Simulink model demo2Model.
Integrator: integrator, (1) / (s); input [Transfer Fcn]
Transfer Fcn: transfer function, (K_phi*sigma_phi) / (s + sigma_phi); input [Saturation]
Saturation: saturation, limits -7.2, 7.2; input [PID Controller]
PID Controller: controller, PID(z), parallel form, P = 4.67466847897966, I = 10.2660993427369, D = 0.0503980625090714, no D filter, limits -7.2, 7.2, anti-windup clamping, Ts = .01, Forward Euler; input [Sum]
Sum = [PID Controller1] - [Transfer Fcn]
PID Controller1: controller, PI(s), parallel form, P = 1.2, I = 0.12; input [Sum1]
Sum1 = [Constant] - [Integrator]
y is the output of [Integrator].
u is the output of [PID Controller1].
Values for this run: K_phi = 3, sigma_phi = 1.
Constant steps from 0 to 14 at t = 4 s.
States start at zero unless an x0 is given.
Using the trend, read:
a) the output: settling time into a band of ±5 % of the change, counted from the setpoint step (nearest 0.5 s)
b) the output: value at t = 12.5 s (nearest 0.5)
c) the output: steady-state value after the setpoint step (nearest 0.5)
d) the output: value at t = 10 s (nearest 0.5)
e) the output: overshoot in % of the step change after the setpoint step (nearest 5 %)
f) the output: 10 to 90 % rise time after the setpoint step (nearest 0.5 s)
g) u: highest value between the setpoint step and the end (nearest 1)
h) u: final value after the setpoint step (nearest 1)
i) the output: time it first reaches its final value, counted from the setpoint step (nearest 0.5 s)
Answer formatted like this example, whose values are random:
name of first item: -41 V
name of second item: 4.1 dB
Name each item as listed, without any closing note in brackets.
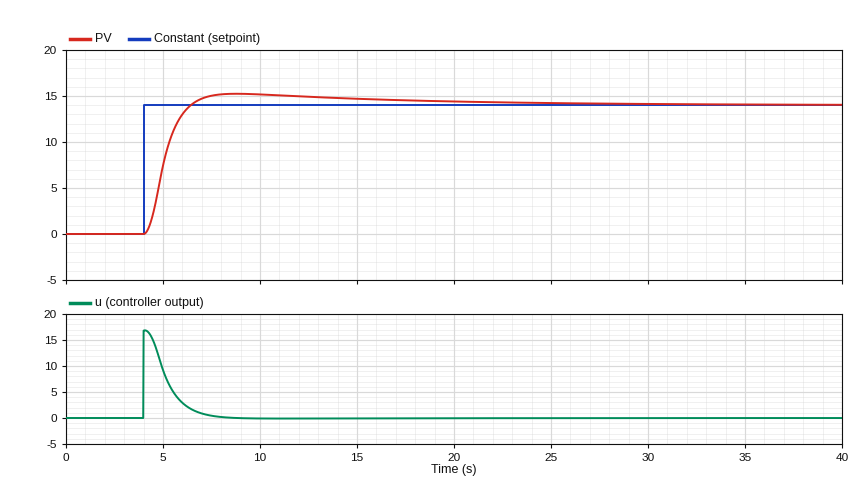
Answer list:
the output: settling time into a band of ±5 % of the change, counted from the setpoint step: 11.0 s
the output: value at t = 12.5 s: 15.0
the output: steady-state value after the setpoint step: 14.0
the output: value at t = 10 s: 15.0
the output: overshoot in % of the step change after the setpoint step: 10 %
the output: 10 to 90 % rise time after the setpoint step: 1.5 s
u: highest value between the setpoint step and the end: 17
u: final value after the setpoint step: 0
the output: time it first reaches its final value, counted from the setpoint step: 2.5 s
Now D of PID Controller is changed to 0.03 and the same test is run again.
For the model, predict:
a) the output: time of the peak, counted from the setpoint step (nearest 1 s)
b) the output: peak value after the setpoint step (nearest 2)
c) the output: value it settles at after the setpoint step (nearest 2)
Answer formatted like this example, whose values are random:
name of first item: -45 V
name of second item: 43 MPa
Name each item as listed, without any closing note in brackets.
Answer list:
the output: time of the peak, counted from the setpoint step: 5 s
the output: peak value after the setpoint step: 16
the output: value it settles at after the setpoint step: 14
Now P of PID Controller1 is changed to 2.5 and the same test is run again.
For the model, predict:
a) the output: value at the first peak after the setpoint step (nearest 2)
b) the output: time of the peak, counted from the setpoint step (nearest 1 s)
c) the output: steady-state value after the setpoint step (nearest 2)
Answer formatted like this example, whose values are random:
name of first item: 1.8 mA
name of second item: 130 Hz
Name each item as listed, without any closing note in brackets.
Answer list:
the output: value at the first peak after the setpoint step: 14
the output: time of the peak, counted from the setpoint step: 4 s
the output: steady-state value after the setpoint step: 14
